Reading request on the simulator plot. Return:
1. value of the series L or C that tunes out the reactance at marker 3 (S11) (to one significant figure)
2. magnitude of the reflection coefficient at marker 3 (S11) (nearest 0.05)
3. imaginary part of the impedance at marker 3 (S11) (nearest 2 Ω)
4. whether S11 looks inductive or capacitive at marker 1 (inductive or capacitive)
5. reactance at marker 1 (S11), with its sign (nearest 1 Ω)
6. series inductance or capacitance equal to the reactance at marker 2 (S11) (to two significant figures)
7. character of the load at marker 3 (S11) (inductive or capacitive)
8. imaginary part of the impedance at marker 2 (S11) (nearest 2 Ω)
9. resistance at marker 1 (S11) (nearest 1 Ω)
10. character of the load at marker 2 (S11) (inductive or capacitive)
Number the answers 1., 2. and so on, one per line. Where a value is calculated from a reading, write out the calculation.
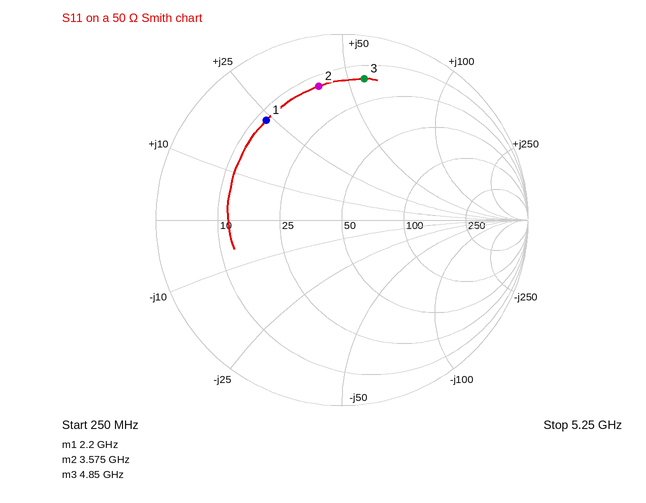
1. C = 1/(2π × 4.85 GHz × 56 Ω) ≈ 586 fF, so 600 fF to one significant figure
2. 0.75
3. +56 Ω
4. inductive
5. +24 Ω
6. L = 40 Ω/(2π × 3.575 GHz) ≈ 1.8 nH
7. inductive
8. +40 Ω
9. 12 Ω
10. inductive
